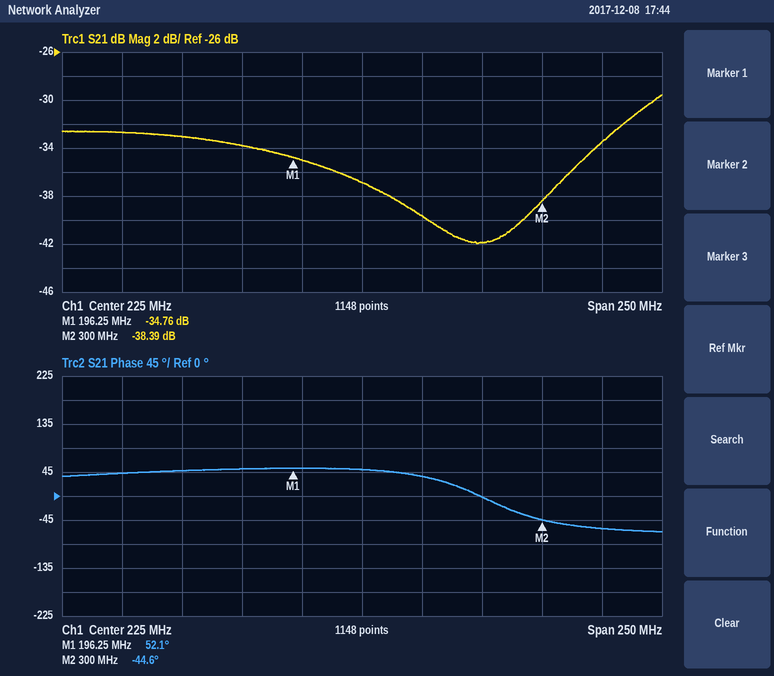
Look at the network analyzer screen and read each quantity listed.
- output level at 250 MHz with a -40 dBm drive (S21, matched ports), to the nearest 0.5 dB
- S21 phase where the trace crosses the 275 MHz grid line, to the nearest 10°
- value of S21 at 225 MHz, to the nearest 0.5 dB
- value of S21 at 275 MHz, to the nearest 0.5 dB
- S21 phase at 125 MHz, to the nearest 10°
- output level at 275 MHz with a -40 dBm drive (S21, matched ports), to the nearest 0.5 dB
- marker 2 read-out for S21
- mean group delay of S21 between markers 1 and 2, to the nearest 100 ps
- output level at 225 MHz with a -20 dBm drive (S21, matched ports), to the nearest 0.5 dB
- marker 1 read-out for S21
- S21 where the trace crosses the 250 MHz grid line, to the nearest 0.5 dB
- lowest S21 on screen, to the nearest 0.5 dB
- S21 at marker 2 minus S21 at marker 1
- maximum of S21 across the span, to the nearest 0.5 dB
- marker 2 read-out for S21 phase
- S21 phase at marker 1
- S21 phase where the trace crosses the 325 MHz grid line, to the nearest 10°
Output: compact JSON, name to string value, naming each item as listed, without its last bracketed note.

{"output level at 250 MHz with a -40 dBm drive (S21, matched ports), to the nearest 0.5 dB": "-79.5 dBm", "S21 phase where the trace crosses the 275 MHz grid line, to the nearest 10°": "0°", "value of S21 at 225 MHz, to the nearest 0.5 dB": "-37.0 dB", "value of S21 at 275 MHz, to the nearest 0.5 dB": "-42.0 dB", "S21 phase at 125 MHz, to the nearest 10°": "40°", "output level at 275 MHz with a -40 dBm drive (S21, matched ports), to the nearest 0.5 dB": "-82.0 dBm", "marker 2 read-out for S21": "-38.39 dB", "mean group delay of S21 between markers 1 and 2, to the nearest 100 ps": "2.6 ns", "output level at 225 MHz with a -20 dBm drive (S21, matched ports), to the nearest 0.5 dB": "-57.0 dBm", "marker 1 read-out for S21": "-34.76 dB", "S21 where the trace crosses the 250 MHz grid line, to the nearest 0.5 dB": "-39.5 dB", "lowest S21 on screen, to the nearest 0.5 dB": "-42.0 dB", "S21 at marker 2 minus S21 at marker 1": "-3.63 dB", "maximum of S21 across the span, to the nearest 0.5 dB": "-29.5 dB", "marker 2 read-out for S21 phase": "-44.6°", "S21 phase at marker 1": "52.1°", "S21 phase where the trace crosses the 325 MHz grid line, to the nearest 10°": "-60°"}
